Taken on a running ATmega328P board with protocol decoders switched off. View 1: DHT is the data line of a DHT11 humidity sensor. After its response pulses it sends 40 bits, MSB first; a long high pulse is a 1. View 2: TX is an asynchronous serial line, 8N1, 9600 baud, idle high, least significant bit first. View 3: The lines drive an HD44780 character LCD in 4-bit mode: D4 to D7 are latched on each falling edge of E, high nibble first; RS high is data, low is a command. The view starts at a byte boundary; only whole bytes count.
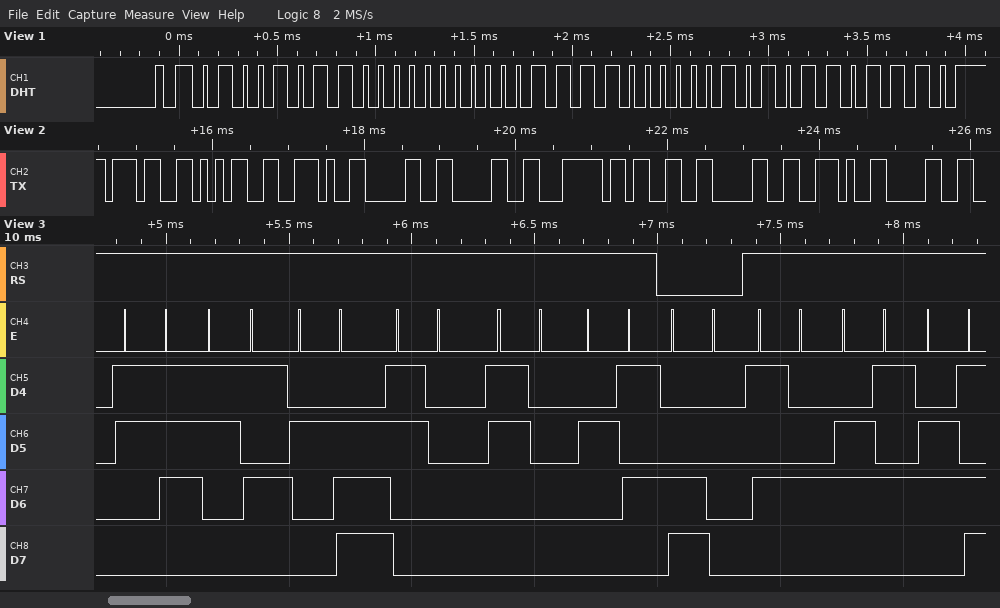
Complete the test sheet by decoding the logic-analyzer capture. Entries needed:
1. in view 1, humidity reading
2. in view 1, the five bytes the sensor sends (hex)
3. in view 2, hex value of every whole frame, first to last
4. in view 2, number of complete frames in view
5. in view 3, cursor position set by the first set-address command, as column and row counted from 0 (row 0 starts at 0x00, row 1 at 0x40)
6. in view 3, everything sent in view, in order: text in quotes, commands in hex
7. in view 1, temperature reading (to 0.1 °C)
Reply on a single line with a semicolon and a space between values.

75 %; 4B 00 1E 05 6E; 0x37 0x35 0x2E 0x30 0x30 0x7C 0x33 0x30 0x2E 0x30; 10; column 0, row 1; "75.00%" 0xC0 "Tem"; 30.5 °C
